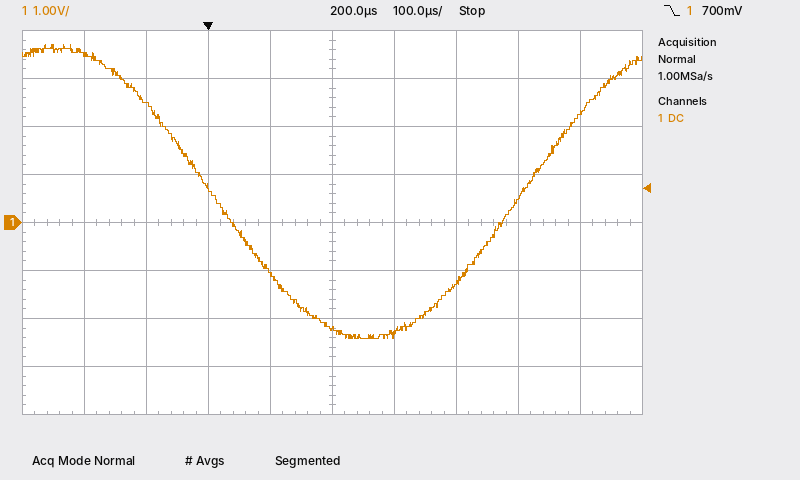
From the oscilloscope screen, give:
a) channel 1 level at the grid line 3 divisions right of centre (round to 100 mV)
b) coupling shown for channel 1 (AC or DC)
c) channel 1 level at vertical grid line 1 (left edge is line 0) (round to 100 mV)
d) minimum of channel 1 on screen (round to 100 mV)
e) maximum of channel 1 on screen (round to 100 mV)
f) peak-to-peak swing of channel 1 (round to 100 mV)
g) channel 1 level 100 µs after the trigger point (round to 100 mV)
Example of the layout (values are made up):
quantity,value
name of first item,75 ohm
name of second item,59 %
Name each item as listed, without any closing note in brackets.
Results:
quantity,value
channel 1 level at the grid line 3 divisions right of centre,500 mV
coupling shown for channel 1,DC
channel 1 level at vertical grid line 1 (left edge is line 0),3.5 V
minimum of channel 1 on screen,-2.4 V
maximum of channel 1 on screen,3.7 V
peak-to-peak swing of channel 1,6.1 V
channel 1 level 100 µs after the trigger point,-1.0 V
